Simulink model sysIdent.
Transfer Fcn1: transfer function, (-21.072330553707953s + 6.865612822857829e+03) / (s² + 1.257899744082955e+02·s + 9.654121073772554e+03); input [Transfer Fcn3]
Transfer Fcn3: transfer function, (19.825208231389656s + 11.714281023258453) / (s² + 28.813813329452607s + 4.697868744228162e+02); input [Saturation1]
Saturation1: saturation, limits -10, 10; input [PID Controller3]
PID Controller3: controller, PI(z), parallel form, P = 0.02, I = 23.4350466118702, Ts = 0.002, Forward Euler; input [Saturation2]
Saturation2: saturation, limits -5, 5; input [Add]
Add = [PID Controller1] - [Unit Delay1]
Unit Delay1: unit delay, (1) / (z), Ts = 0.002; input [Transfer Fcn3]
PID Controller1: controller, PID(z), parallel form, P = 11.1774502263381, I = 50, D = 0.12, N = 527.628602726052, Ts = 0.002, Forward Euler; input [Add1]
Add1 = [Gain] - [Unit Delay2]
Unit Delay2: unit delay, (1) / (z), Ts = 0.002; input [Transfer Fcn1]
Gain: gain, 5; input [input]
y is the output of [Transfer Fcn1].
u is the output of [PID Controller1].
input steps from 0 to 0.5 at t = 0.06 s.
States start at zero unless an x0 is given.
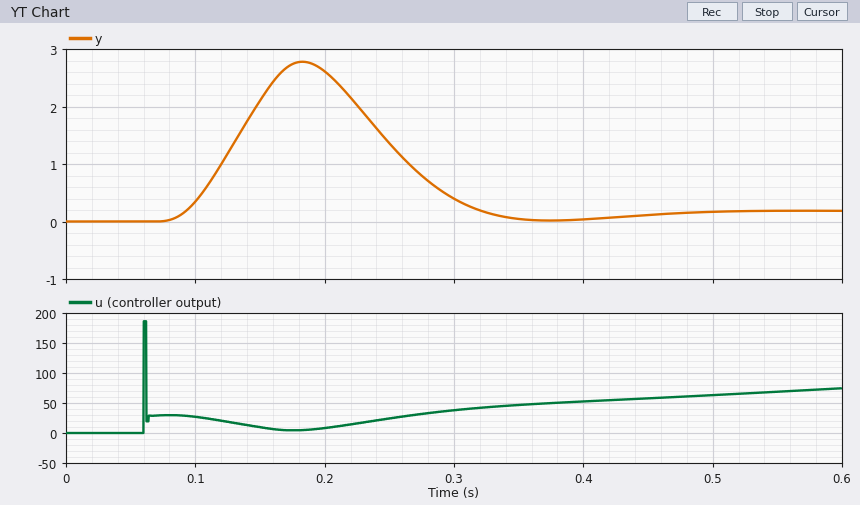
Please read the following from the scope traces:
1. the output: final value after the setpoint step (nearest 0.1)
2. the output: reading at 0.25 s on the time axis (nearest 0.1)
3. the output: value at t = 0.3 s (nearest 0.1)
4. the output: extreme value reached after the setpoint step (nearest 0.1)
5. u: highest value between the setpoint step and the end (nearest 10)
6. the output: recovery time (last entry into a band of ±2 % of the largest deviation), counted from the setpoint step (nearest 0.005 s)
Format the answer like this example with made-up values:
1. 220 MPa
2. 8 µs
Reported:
1. 0.2
2. 1.4
3. 0.4
4. 2.8
5. 190
6. 0.395 s
